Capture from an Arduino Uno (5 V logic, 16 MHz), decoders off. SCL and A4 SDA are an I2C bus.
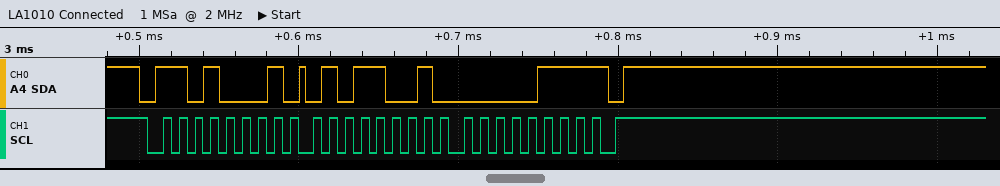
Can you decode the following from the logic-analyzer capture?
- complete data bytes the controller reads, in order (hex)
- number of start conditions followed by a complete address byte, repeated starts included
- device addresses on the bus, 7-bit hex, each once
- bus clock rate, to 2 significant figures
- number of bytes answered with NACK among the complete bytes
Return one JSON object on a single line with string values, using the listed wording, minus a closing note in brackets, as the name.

{"complete data bytes the controller reads, in order": "59 07", "number of start conditions followed by a complete address byte, repeated starts included": "1", "device addresses on the bus, 7-bit hex, each once": "0x68", "bus clock rate, to 2 significant figures": "100 kHz", "number of bytes answered with NACK among the complete bytes": "1"}
